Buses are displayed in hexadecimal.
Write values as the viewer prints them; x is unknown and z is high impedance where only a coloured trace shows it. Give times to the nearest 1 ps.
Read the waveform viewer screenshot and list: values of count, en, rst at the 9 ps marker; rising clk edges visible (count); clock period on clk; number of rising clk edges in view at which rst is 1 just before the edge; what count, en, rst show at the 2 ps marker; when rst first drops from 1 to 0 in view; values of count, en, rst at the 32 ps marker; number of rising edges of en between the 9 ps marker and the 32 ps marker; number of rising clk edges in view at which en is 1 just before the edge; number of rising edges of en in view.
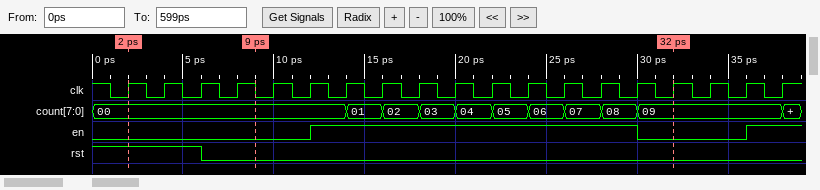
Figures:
count=00, en=0, rst=0
19
2 ps
3
count=00, en=0, rst=1
6 ps
count=09, en=0, rst=0
1
10
2
